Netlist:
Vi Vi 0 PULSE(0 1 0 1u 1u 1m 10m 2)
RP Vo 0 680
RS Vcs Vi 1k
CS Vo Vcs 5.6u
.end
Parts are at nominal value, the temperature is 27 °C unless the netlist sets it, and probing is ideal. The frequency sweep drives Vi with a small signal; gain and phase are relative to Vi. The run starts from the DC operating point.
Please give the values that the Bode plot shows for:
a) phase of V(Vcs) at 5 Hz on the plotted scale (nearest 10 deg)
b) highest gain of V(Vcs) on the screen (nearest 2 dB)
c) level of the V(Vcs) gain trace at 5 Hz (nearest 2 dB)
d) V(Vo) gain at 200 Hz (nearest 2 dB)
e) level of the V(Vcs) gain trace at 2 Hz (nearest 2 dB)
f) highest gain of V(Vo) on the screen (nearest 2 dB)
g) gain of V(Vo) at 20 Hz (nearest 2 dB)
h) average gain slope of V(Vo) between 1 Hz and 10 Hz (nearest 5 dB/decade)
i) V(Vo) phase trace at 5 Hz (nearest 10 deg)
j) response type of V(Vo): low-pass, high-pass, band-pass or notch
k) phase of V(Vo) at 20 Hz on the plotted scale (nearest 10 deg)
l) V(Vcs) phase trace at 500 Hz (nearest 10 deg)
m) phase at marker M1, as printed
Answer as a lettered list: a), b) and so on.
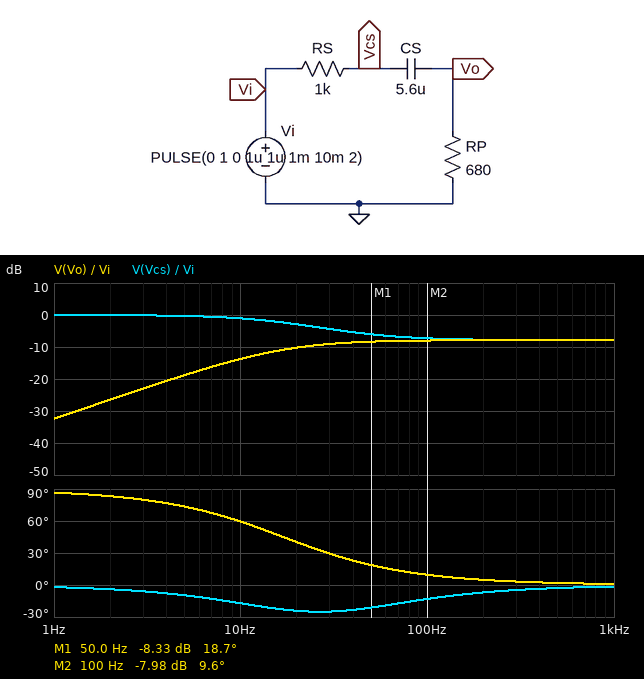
a) -10 deg
b) 0 dB
c) 0 dB
d) -8 dB
e) 0 dB
f) -8 dB
g) -10 dB
h) 20 dB/decade
i) 70 deg
j) high-pass
k) 40 deg
l) 0 deg
m) 18.7 deg
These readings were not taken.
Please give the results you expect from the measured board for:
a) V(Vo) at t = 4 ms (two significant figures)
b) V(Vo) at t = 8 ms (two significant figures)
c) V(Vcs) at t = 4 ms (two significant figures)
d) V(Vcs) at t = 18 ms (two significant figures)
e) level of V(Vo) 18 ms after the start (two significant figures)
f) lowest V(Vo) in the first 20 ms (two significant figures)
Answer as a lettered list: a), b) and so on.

a) -30 mV
b) -19 mV
c) 44 mV
d) 38 mV
e) -26 mV
f) -55 mV
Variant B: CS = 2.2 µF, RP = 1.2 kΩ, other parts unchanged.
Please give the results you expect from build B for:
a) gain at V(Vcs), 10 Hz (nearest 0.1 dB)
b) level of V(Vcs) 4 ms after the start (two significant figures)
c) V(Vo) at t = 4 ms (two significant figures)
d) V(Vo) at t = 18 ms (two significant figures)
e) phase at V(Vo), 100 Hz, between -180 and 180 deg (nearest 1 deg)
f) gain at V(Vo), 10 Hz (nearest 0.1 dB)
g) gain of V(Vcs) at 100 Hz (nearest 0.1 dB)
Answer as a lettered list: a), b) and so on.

a) -0.3 dB
b) 46 mV
c) -55 mV
d) -27 mV
e) 18 deg
f) -16.0 dB
g) -4.4 dB
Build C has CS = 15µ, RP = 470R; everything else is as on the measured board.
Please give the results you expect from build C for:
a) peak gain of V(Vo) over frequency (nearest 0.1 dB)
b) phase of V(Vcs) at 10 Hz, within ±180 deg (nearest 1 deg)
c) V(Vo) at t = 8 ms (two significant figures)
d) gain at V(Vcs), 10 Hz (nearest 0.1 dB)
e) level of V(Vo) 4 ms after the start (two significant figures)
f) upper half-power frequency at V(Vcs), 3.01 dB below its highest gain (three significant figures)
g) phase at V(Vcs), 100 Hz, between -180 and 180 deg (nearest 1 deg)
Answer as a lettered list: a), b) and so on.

a) -9.9 dB
b) -30 deg
c) -10 mV
d) -3.9 dB
e) -12 mV
f) 8.09 Hz
g) -9 deg
